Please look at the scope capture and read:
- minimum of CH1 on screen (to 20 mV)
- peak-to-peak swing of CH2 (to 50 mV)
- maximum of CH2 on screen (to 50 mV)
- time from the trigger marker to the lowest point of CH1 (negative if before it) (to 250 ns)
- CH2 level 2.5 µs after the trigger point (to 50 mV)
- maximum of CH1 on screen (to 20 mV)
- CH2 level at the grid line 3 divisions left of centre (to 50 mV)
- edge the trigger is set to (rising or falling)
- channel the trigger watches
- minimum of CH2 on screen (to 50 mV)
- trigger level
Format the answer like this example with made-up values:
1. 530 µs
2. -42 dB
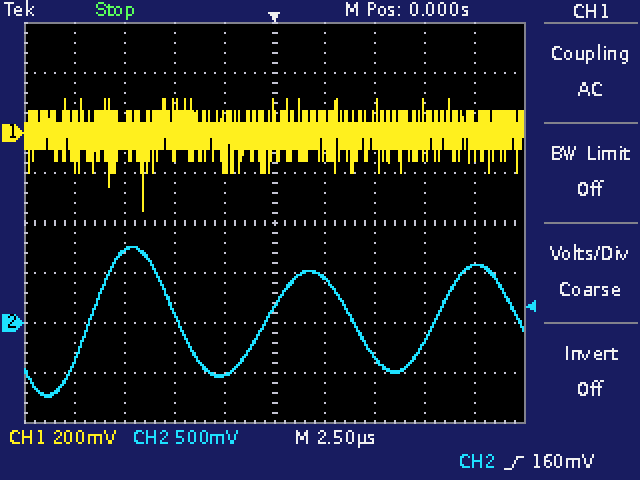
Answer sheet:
1. -320 mV
2. 1.50 V
3. 750 mV
4. -6.50 µs
5. 450 mV
6. 140 mV
7. 700 mV
8. rising
9. CH2
10. -750 mV
11. 160 mV
